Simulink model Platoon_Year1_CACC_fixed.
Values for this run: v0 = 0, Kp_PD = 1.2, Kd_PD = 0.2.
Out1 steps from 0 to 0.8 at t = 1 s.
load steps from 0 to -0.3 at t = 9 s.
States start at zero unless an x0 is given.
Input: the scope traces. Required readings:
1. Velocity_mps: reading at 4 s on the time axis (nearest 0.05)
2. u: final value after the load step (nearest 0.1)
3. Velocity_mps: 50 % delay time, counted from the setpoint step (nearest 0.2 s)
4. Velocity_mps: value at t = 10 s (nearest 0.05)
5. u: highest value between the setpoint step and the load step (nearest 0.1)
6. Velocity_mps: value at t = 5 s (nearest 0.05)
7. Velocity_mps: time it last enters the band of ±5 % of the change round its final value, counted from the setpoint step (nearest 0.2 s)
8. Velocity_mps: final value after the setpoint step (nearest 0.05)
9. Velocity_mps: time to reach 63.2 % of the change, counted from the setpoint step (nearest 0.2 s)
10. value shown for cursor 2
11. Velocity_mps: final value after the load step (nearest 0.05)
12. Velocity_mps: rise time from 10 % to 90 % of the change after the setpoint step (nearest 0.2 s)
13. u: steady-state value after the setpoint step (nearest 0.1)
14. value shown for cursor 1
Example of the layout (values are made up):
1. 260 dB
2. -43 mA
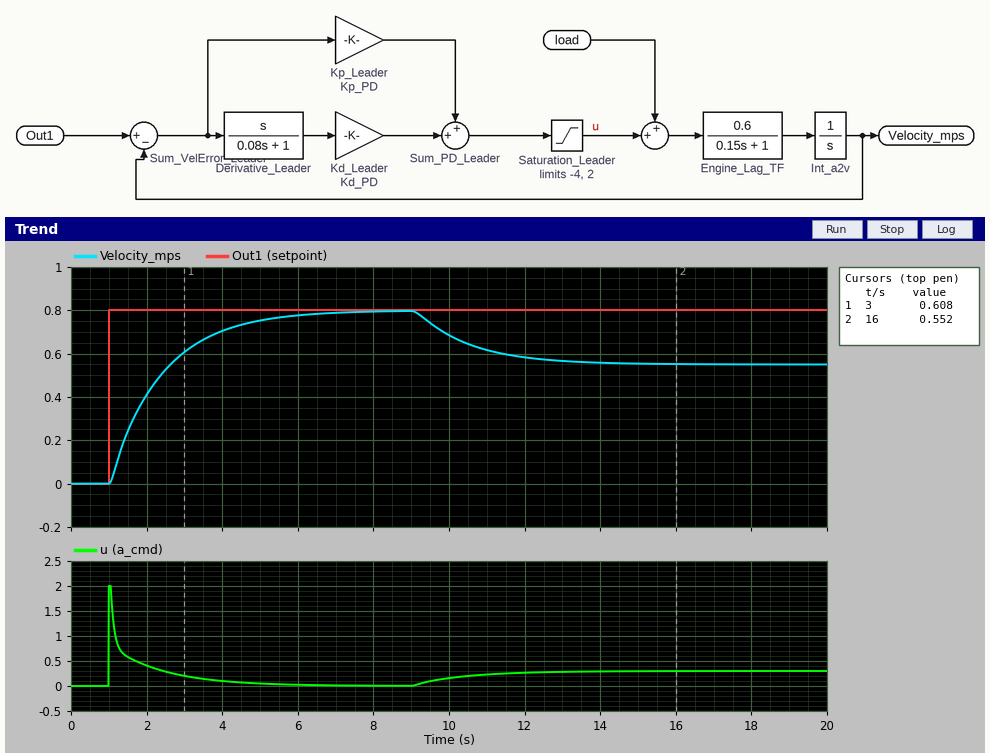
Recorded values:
1. 0.70
2. 0.3
3. 1.0 s
4. 0.70
5. 2.0
6. 0.75
7. 4.2 s
8. 0.80
9. 1.4 s
10. 0.552
11. 0.55
12. 3.0 s
13. 0.0
14. 0.608
